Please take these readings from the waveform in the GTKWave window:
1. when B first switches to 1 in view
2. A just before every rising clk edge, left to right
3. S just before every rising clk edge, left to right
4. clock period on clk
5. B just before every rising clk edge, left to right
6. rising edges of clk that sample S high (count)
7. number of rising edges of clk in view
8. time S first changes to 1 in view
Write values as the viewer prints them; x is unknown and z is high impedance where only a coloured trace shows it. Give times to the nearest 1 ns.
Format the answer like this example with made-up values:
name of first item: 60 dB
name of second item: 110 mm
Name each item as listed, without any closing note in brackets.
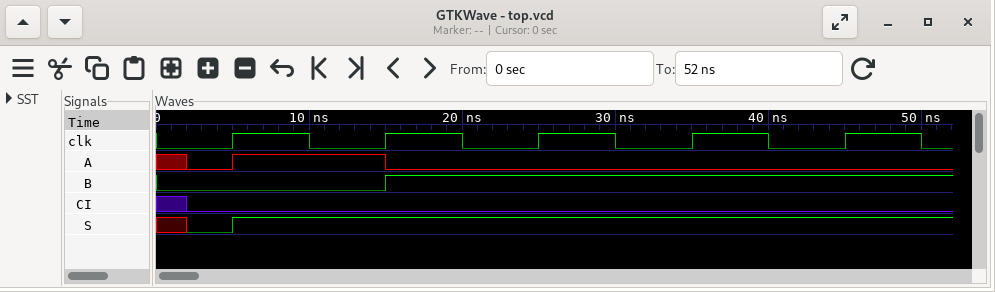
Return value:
when B first switches to 1 in view: 15 ns
A just before every rising clk edge, left to right: 0 1 0 0 0
S just before every rising clk edge, left to right: 0 1 1 1 1
clock period on clk: 10 ns
B just before every rising clk edge, left to right: 0 0 1 1 1
rising edges of clk that sample S high: 4
number of rising edges of clk in view: 5
time S first changes to 1 in view: 5 ns
